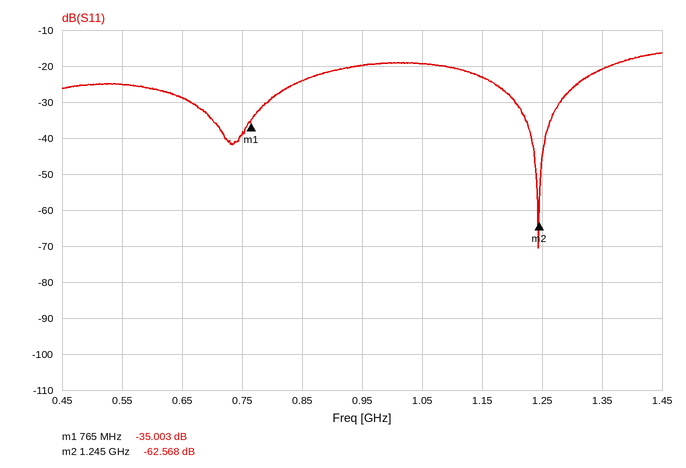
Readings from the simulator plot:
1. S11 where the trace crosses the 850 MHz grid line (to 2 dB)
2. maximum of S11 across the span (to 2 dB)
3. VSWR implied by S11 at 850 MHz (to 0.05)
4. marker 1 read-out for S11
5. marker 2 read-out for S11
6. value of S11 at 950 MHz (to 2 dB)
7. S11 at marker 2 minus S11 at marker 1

-24 dB
-16 dB
1.15
-35.003 dB
-62.568 dB
-20 dB
-27.565 dB
